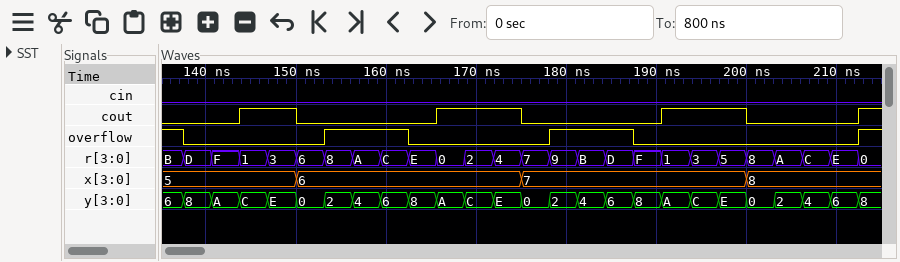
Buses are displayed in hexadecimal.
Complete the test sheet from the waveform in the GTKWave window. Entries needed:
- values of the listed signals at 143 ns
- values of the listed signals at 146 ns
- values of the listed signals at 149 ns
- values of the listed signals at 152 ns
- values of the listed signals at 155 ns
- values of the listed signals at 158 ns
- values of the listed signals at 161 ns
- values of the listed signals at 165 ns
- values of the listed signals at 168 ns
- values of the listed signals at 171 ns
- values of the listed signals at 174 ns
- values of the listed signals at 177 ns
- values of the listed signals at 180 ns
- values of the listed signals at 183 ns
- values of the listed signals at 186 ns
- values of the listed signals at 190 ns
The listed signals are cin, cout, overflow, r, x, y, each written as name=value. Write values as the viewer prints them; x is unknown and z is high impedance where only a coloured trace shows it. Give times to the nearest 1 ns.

cin=0, cout=0, overflow=0, r=F, x=5, y=A
cin=0, cout=1, overflow=0, r=1, x=5, y=C
cin=0, cout=1, overflow=0, r=3, x=5, y=E
cin=0, cout=0, overflow=0, r=6, x=6, y=0
cin=0, cout=0, overflow=1, r=8, x=6, y=2
cin=0, cout=0, overflow=1, r=A, x=6, y=4
cin=0, cout=0, overflow=1, r=C, x=6, y=6
cin=0, cout=0, overflow=0, r=E, x=6, y=8
cin=0, cout=1, overflow=0, r=0, x=6, y=A
cin=0, cout=1, overflow=0, r=2, x=6, y=C
cin=0, cout=1, overflow=0, r=4, x=6, y=E
cin=0, cout=0, overflow=0, r=7, x=7, y=0
cin=0, cout=0, overflow=1, r=9, x=7, y=2
cin=0, cout=0, overflow=1, r=B, x=7, y=4
cin=0, cout=0, overflow=1, r=D, x=7, y=6
cin=0, cout=0, overflow=0, r=F, x=7, y=8
